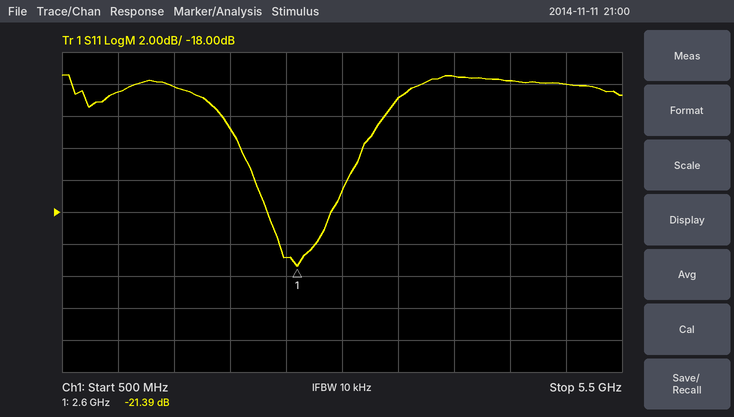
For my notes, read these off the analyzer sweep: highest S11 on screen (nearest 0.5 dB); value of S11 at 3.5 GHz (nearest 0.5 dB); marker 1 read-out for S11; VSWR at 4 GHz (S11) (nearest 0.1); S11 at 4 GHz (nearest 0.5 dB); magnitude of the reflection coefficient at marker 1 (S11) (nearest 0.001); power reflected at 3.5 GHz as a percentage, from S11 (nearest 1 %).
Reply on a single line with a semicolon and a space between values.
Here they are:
-9.5 dB; -11.0 dB; -21.39 dB; 2.0; -9.5 dB; 0.085; 8 %
